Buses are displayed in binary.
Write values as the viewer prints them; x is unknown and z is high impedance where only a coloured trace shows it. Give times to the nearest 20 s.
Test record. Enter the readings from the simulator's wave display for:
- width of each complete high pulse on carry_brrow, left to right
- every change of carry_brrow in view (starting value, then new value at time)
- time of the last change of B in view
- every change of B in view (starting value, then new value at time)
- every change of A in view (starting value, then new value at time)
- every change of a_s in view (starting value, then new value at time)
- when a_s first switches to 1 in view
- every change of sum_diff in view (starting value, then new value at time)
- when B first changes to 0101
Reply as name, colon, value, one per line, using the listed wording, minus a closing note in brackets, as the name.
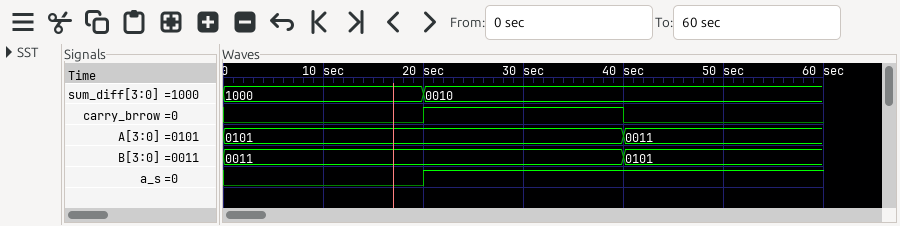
width of each complete high pulse on carry_brrow, left to right: 20 s
every change of carry_brrow in view: 0, 1 at 20 s, 0 at 40 s
time of the last change of B in view: 40 s
every change of B in view: 0011, 0101 at 40 s
every change of A in view: 0101, 0011 at 40 s
every change of a_s in view: 0, 1 at 20 s
when a_s first switches to 1 in view: 20 s
every change of sum_diff in view: 1000, 0010 at 20 s
when B first changes to 0101: 40 s
